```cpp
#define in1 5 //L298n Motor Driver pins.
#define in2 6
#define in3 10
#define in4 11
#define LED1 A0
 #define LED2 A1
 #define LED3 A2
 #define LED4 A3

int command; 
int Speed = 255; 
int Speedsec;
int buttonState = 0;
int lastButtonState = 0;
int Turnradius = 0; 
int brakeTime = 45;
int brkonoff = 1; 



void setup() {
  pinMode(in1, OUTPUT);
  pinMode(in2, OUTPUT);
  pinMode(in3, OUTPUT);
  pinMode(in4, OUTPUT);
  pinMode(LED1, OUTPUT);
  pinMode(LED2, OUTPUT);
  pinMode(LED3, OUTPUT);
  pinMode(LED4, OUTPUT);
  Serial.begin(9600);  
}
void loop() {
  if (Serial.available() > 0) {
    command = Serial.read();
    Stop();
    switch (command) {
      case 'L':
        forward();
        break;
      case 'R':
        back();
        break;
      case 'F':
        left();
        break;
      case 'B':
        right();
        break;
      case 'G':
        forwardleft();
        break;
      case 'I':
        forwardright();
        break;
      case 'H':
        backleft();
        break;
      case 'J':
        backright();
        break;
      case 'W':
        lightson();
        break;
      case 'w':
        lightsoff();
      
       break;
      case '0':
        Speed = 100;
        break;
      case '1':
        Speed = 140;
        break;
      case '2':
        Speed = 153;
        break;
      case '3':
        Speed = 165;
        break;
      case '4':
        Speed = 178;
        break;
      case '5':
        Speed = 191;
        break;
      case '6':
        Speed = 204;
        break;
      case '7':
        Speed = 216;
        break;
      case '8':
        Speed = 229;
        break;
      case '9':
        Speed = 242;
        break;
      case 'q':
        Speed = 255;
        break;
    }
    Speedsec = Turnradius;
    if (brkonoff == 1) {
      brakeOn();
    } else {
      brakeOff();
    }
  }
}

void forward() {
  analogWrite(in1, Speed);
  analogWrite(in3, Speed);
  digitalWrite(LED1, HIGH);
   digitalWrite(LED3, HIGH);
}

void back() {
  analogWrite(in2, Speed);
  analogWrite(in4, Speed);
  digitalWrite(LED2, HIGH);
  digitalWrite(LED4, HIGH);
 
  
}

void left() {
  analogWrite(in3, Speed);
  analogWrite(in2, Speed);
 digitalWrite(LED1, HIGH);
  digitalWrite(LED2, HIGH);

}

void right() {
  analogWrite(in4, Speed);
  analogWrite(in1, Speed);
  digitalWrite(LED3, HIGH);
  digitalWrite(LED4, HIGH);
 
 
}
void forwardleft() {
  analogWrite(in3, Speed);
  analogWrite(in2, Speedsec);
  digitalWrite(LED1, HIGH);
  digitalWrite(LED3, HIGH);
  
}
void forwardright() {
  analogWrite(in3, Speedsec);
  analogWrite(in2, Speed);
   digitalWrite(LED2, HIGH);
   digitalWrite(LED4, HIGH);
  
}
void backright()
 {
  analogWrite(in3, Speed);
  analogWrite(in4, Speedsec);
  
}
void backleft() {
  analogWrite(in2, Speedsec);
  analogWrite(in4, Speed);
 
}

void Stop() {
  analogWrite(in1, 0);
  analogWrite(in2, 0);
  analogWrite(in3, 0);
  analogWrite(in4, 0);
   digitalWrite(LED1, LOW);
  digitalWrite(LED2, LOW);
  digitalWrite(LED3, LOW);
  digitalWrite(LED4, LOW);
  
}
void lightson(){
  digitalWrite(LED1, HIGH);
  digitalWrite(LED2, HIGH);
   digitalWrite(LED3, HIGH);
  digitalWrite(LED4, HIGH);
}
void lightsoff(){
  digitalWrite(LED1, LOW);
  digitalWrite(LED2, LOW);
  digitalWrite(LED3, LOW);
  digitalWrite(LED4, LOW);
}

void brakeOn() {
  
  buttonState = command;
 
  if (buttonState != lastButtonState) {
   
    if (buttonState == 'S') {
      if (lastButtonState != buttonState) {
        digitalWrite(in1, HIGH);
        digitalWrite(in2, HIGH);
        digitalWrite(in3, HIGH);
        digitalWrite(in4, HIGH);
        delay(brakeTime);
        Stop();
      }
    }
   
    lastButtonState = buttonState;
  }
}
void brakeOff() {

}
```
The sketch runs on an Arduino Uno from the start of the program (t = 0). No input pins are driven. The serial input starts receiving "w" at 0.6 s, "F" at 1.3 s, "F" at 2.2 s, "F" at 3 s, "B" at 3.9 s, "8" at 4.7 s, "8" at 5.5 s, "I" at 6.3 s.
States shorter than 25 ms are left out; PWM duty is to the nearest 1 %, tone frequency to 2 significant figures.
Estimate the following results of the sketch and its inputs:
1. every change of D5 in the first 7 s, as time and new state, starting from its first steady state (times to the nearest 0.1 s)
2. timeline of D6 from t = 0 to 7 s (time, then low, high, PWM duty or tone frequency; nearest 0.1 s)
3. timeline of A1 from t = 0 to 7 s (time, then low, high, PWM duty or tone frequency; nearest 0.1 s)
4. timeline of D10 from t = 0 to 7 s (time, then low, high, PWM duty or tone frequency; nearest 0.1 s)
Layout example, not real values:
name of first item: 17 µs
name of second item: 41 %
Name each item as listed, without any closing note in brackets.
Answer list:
every change of D5 in the first 7 s, as time and new state, starting from its first steady state: 0 s low; 3.9 s high; 4.7 s low
timeline of D6 from t = 0 to 7 s: 0 s low; 1.3 s high; 3.9 s low; 6.3 s PWM 90 %
timeline of A1 from t = 0 to 7 s: 0 s low; 1.3 s high; 3.9 s low; 6.3 s high
timeline of D10 from t = 0 to 7 s: 0 s low; 1.3 s high; 3.9 s low
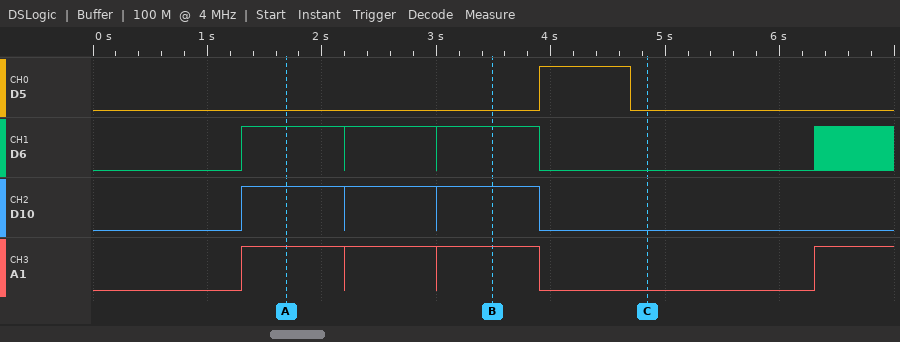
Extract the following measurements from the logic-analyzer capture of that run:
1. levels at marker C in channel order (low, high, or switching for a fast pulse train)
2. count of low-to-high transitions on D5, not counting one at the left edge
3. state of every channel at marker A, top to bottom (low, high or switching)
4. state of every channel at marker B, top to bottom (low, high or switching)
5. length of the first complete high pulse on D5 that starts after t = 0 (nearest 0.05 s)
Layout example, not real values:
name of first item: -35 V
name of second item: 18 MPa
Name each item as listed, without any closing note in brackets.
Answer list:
levels at marker C in channel order: D5 low, D6 low, D10 low, A1 low
count of low-to-high transitions on D5, not counting one at the left edge: 1
state of every channel at marker A, top to bottom: D5 low, D6 high, D10 high, A1 high
state of every channel at marker B, top to bottom: D5 low, D6 high, D10 high, A1 high
length of the first complete high pulse on D5 that starts after t = 0: 0.80 s
